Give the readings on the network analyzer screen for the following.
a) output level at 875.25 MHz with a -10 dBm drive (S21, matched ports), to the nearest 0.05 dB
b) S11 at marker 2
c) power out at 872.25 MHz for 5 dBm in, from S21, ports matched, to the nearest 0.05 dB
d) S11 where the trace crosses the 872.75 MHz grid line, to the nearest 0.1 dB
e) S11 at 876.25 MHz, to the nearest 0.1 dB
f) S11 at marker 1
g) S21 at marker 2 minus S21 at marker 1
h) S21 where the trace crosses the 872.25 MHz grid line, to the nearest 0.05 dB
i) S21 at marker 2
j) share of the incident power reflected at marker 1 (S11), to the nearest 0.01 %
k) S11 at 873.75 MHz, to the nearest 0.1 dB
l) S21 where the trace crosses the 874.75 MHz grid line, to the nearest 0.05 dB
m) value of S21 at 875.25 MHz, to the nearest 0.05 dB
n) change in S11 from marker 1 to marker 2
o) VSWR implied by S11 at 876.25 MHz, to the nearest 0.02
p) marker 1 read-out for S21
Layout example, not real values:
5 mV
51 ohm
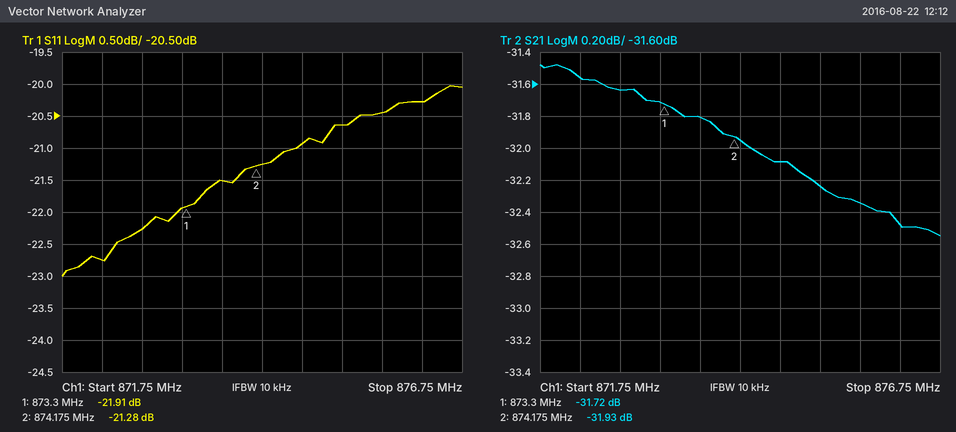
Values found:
-42.25 dBm
-21.28 dB
-26.55 dBm
-22.3 dB
-20.3 dB
-21.91 dB
-0.21 dB
-31.55 dB
-31.93 dB
0.64 %
-21.5 dB
-32.10 dB
-32.25 dB
0.63 dB
1.22
-31.72 dB
